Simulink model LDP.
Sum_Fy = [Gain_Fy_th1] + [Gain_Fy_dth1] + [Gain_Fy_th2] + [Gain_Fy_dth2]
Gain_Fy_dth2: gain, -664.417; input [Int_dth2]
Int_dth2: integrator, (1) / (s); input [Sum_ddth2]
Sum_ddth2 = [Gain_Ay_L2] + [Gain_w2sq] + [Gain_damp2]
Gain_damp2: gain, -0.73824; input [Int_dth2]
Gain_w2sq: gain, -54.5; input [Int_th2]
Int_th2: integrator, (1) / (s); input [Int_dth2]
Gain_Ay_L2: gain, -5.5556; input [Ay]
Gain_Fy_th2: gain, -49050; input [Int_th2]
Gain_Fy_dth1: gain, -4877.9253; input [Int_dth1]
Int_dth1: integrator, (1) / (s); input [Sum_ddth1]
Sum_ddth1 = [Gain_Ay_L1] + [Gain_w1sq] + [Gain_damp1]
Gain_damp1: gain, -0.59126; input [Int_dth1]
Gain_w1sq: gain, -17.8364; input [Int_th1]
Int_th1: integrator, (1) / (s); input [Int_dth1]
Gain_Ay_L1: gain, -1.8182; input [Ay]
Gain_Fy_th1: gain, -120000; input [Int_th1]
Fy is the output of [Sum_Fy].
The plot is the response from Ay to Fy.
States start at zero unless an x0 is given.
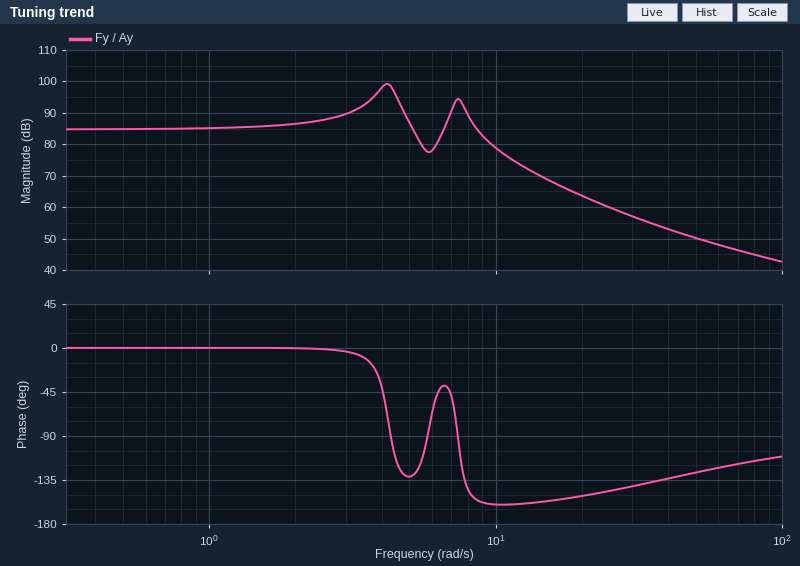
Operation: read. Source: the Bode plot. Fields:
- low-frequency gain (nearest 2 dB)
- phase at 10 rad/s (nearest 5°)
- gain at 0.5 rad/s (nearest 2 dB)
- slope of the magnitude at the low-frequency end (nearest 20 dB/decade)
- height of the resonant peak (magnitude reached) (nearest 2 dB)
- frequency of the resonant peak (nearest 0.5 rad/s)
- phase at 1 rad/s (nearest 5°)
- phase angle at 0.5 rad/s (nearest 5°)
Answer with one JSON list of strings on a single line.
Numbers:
["84 dB", "-160°", "84 dB", "0 dB/decade", "100 dB", "4.0 rad/s", "0°", "0°"]
